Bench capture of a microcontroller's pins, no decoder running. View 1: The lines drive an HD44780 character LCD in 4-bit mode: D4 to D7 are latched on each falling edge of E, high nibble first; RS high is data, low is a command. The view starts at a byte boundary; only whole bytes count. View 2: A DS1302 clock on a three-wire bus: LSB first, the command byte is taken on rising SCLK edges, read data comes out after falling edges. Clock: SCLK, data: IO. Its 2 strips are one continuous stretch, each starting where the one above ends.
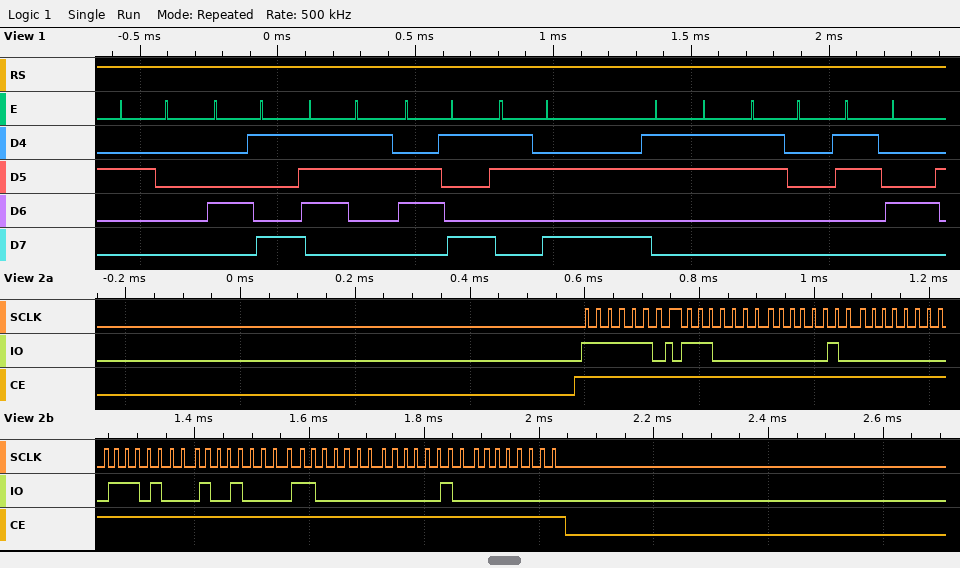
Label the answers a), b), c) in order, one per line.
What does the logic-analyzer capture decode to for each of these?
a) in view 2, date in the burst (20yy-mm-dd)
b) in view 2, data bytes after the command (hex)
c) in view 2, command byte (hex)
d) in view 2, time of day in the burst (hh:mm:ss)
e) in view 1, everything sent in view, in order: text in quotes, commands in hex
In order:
a) 2020-09-17
b) 07 20 00 17 09 03 20 00
c) 0xBF
d) 00:20:07
e) " Isi:304"
